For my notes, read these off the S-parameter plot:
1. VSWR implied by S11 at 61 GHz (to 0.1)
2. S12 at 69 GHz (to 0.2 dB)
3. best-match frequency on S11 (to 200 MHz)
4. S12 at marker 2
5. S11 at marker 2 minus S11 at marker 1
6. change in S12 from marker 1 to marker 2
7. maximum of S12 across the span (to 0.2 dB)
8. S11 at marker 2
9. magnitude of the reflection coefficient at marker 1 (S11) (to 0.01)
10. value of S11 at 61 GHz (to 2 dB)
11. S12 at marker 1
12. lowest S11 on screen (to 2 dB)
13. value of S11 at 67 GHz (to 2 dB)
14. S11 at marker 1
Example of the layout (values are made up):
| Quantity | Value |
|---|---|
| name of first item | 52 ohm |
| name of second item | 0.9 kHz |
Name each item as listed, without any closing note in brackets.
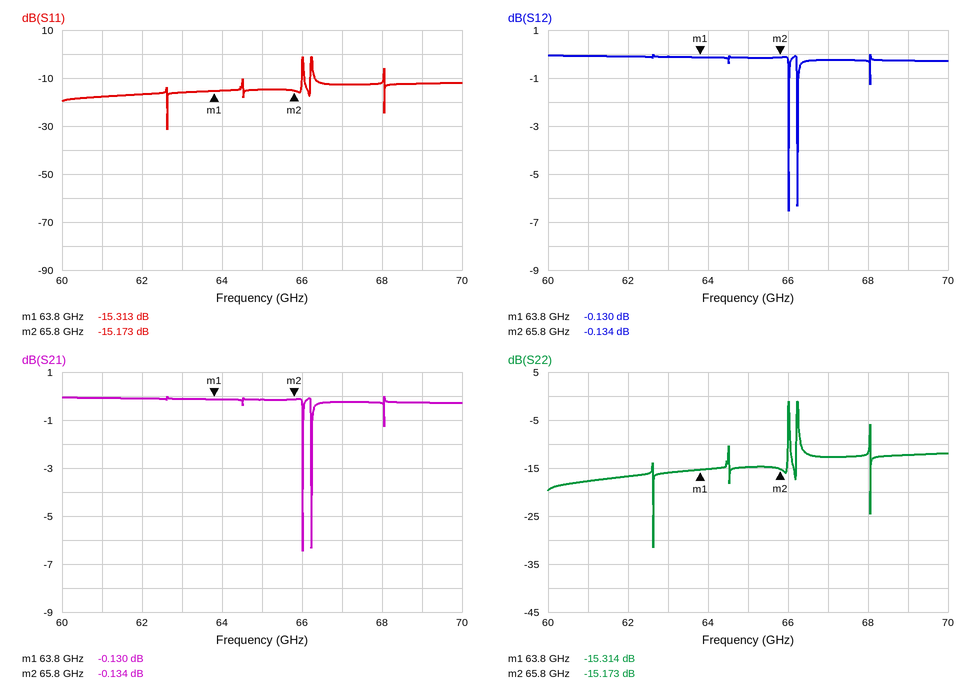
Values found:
| Quantity | Value |
|---|---|
| VSWR implied by S11 at 61 GHz | 1.3 |
| S12 at 69 GHz | -0.2 dB |
| best-match frequency on S11 | 62.6 GHz |
| S12 at marker 2 | -0.134 dB |
| S11 at marker 2 minus S11 at marker 1 | 0.140 dB |
| change in S12 from marker 1 to marker 2 | -0.004 dB |
| maximum of S12 across the span | 0.0 dB |
| S11 at marker 2 | -15.173 dB |
| magnitude of the reflection coefficient at marker 1 (S11) | 0.17 |
| value of S11 at 61 GHz | -18 dB |
| S12 at marker 1 | -0.130 dB |
| lowest S11 on screen | -32 dB |
| value of S11 at 67 GHz | -12 dB |
| S11 at marker 1 | -15.313 dB |
